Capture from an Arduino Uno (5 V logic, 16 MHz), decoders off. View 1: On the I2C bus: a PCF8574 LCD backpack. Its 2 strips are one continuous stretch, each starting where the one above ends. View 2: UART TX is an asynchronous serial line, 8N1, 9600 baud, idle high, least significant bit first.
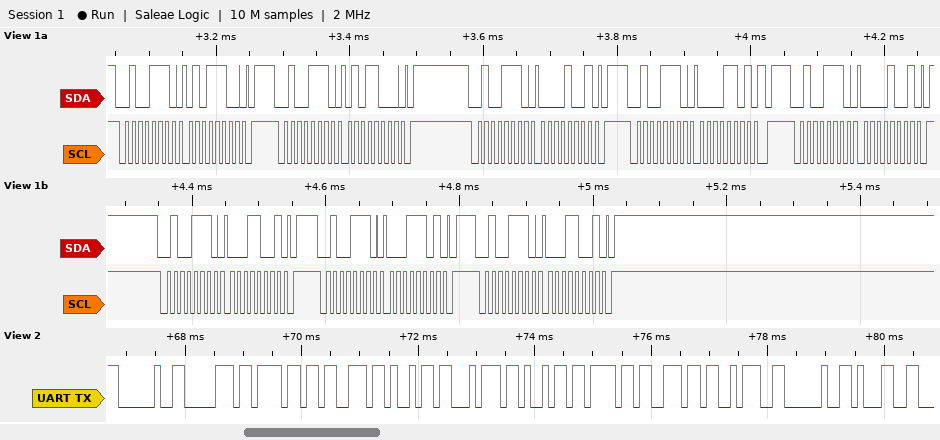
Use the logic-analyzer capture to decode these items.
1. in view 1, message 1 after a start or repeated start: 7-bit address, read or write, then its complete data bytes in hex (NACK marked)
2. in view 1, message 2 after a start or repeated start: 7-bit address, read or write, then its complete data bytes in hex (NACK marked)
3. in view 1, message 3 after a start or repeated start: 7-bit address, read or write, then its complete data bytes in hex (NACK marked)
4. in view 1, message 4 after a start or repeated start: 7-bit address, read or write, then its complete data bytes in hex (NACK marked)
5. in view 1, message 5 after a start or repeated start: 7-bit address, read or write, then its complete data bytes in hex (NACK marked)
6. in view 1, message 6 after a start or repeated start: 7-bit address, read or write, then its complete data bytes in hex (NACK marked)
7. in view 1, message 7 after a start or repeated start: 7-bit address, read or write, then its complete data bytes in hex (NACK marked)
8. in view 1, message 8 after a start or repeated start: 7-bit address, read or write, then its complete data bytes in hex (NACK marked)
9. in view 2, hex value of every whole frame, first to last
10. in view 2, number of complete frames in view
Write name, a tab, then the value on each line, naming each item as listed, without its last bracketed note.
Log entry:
in view 1, message 1 after a start or repeated start: 7-bit address, read or write, then its complete data bytes in hex	0x27 write: 5C
in view 1, message 2 after a start or repeated start: 7-bit address, read or write, then its complete data bytes in hex	0x27 write: 58
in view 1, message 3 after a start or repeated start: 7-bit address, read or write, then its complete data bytes in hex	0x27 write: 09
in view 1, message 4 after a start or repeated start: 7-bit address, read or write, then its complete data bytes in hex	0x27 write: 0D
in view 1, message 5 after a start or repeated start: 7-bit address, read or write, then its complete data bytes in hex	0x27 write: 09
in view 1, message 6 after a start or repeated start: 7-bit address, read or write, then its complete data bytes in hex	0x27 write: 19
in view 1, message 7 after a start or repeated start: 7-bit address, read or write, then its complete data bytes in hex	0x27 write: 1D
in view 1, message 8 after a start or repeated start: 7-bit address, read or write, then its complete data bytes in hex	0x27 write: 19
in view 2, hex value of every whole frame, first to last	20 70 6F 73 69 74 69 6F 6E 3A 20 31
in view 2, number of complete frames in view	12
